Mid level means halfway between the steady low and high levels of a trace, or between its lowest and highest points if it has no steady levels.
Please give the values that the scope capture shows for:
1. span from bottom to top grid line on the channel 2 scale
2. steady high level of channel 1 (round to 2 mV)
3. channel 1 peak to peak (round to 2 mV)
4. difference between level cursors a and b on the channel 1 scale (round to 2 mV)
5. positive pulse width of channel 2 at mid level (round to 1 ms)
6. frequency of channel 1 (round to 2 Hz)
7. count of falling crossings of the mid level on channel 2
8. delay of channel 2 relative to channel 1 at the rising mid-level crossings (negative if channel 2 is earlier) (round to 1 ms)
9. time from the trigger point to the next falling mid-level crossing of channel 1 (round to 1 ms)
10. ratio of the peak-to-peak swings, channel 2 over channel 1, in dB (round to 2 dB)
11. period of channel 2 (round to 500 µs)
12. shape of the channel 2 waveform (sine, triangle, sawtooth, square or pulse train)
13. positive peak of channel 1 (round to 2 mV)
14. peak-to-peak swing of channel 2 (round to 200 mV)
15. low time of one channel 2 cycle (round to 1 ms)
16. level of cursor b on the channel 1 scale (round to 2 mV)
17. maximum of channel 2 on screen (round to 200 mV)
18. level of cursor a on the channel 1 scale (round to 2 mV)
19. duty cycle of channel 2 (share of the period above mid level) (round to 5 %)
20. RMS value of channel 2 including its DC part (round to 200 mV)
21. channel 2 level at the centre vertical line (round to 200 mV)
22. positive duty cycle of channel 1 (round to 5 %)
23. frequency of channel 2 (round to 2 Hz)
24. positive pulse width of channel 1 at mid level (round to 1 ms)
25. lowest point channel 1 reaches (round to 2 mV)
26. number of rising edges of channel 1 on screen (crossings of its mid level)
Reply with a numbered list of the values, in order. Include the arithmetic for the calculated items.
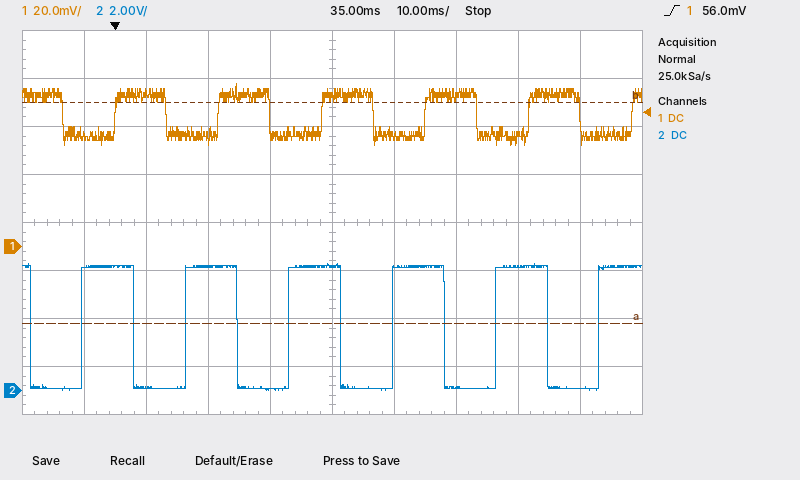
1. 16 V
2. 64 mV
3. 68 mV − (42 mV) = 26 mV
4. 92 mV
5. 8 ms
6. 1 / 16.5 ms ≈ 60.6 Hz, so 60 Hz to the nearest 2 Hz
7. 6
8. -5 ms
9. 8 ms
10. 20 log10(5.2 V / 26 mV) ≈ 46 dB
11. 16.5 ms
12. square
13. 68 mV
14. 5.2 V − (0.0 V) = 5.2 V
15. 8 ms
16. 60 mV
17. 5.2 V
18. -32 mV
19. 8 ms / 16.5 ms ≈ 48.5 %, so 50 % to the nearest 5 %
20. √(0.5 × (5.2 V)² + 0.5 × (0.0 V)²) ≈ 3.68 V, so 3.6 V to the nearest 200 mV
21. 5.2 V
22. 8 ms / 16.5 ms ≈ 48.5 %, so 50 % to the nearest 5 %
23. 1 / 16.5 ms ≈ 60.6 Hz, so 60 Hz to the nearest 2 Hz
24. 8 ms
25. 42 mV
26. 6
